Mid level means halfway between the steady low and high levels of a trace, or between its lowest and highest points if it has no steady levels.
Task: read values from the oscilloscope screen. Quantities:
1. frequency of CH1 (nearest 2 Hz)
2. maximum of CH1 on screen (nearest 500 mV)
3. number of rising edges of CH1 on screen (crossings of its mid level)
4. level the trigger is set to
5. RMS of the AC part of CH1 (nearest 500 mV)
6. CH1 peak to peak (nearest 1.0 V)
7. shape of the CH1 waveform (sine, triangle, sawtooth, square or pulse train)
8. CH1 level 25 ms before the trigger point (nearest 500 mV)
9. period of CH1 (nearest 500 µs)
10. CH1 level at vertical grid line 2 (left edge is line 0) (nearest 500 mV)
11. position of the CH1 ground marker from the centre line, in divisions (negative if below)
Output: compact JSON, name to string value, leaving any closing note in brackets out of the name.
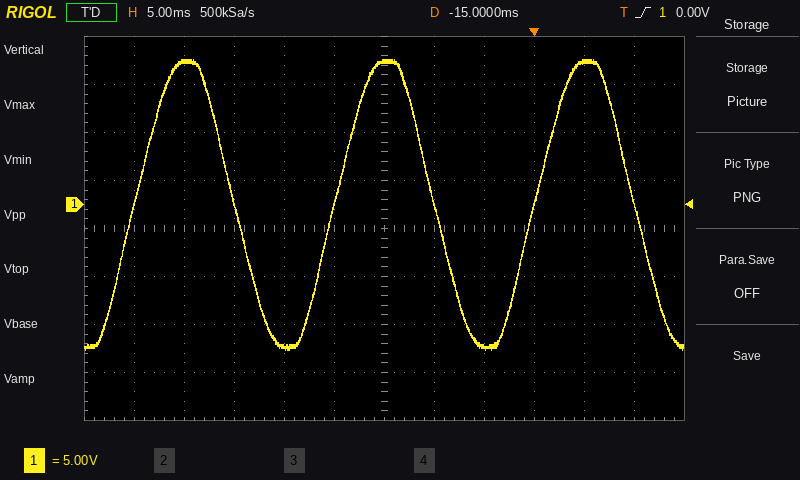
{"frequency of CH1": "50 Hz", "maximum of CH1 on screen": "15.0 V", "number of rising edges of CH1 on screen": "3", "level the trigger is set to": "0.00 V", "RMS of the AC part of CH1": "10.5 V", "CH1 peak to peak": "30.0 V", "shape of the CH1 waveform": "sine", "CH1 level 25 ms before the trigger point": "-15.0 V", "period of CH1": "20.0 ms", "CH1 level at vertical grid line 2 (left edge is line 0)": "15.0 V", "position of the CH1 ground marker from the centre line, in divisions": "+0.5 div"}
